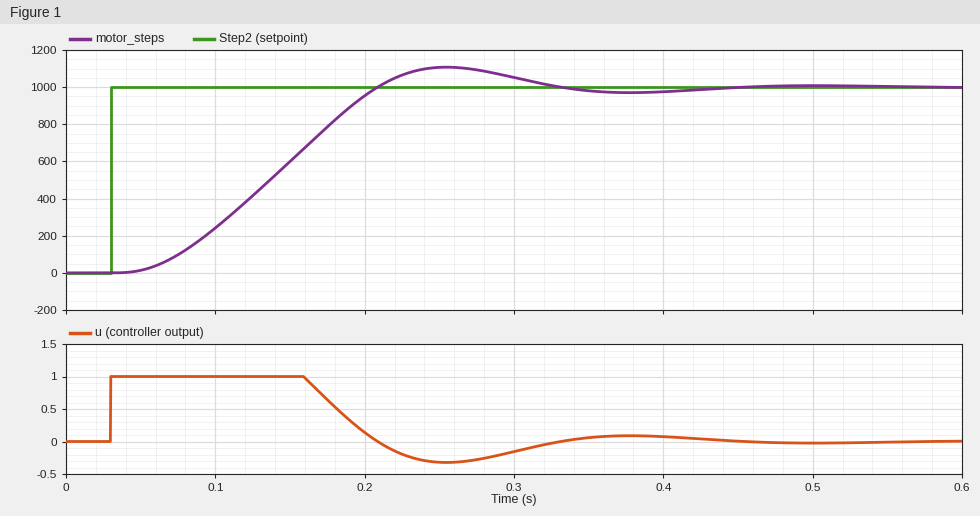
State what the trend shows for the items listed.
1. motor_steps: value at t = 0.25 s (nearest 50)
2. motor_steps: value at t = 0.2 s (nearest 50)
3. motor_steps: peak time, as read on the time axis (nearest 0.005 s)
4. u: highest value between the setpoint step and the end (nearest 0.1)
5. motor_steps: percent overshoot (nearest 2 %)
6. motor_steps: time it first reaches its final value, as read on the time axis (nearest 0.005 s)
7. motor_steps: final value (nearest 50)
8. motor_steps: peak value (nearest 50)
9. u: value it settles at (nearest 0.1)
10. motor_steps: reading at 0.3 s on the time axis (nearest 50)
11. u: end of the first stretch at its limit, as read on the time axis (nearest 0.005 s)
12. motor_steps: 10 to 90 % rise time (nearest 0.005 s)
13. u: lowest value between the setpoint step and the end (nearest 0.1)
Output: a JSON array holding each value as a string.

["1100", "950", "0.255 s", "1.0", "10 %", "0.210 s", "1000", "1100", "0.0", "1050", "0.160 s", "0.115 s", "-0.3"]
